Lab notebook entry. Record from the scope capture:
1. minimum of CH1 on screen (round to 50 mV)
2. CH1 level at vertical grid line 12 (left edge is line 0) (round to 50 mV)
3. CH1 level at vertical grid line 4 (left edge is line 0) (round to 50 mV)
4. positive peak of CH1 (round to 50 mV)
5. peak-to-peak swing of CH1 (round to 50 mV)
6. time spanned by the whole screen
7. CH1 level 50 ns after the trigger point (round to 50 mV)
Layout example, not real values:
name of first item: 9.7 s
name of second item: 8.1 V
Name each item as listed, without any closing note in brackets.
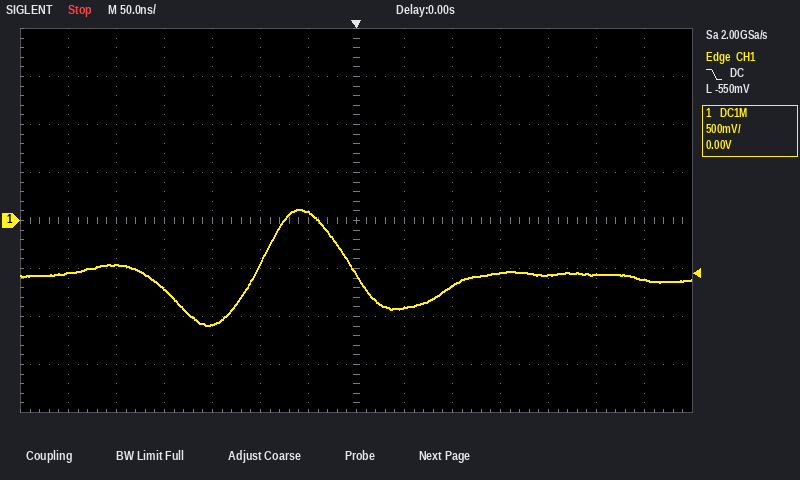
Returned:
minimum of CH1 on screen: -1.10 V
CH1 level at vertical grid line 12 (left edge is line 0): -550 mV
CH1 level at vertical grid line 4 (left edge is line 0): -1.10 V
positive peak of CH1: 100 mV
peak-to-peak swing of CH1: 1.20 V
time spanned by the whole screen: 700 ns
CH1 level 50 ns after the trigger point: -900 mV
